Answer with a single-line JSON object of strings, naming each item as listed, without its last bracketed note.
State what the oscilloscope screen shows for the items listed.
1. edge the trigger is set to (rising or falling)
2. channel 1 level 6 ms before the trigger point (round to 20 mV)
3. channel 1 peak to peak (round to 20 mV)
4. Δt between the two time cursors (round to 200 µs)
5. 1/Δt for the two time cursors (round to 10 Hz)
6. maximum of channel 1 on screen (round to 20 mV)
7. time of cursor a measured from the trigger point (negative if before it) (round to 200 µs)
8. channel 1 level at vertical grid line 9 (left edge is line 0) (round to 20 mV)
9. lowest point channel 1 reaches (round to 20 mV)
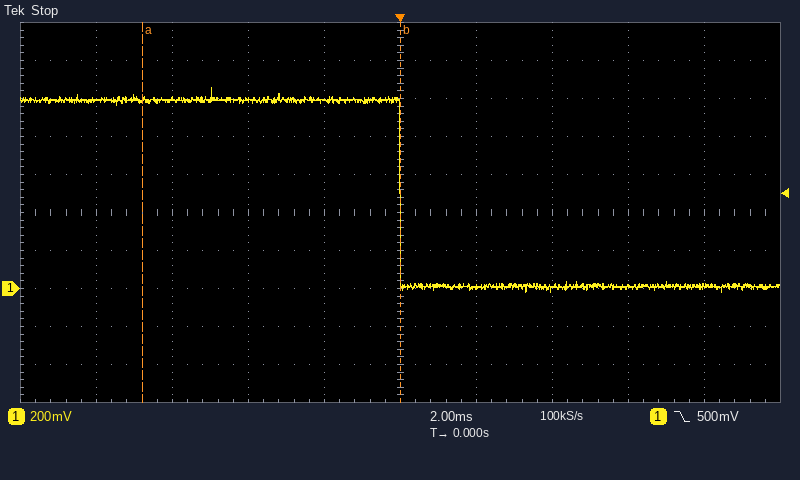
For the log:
{"edge the trigger is set to": "falling", "channel 1 level 6 ms before the trigger point": "1.00 V", "channel 1 peak to peak": "1.08 V", "Δt between the two time cursors": "6.8 ms", "1/Δt for the two time cursors": "150 Hz", "maximum of channel 1 on screen": "1.06 V", "time of cursor a measured from the trigger point (negative if before it)": "-6.8 ms", "channel 1 level at vertical grid line 9 (left edge is line 0)": "20 mV", "lowest point channel 1 reaches": "-20 mV"}
